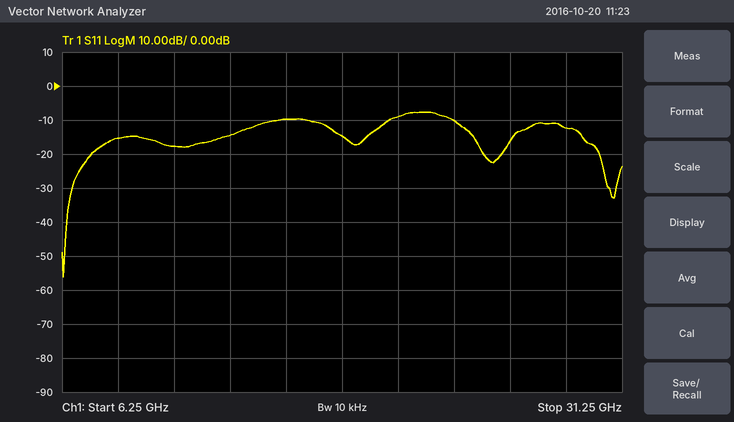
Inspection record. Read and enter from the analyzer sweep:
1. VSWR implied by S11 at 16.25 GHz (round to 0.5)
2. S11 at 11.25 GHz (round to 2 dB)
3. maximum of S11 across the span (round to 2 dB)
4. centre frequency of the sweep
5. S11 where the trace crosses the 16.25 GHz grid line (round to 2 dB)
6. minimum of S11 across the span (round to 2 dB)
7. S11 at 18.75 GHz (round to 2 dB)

2.0
-18 dB
-8 dB
18.75 GHz
-10 dB
-56 dB
-14 dB
